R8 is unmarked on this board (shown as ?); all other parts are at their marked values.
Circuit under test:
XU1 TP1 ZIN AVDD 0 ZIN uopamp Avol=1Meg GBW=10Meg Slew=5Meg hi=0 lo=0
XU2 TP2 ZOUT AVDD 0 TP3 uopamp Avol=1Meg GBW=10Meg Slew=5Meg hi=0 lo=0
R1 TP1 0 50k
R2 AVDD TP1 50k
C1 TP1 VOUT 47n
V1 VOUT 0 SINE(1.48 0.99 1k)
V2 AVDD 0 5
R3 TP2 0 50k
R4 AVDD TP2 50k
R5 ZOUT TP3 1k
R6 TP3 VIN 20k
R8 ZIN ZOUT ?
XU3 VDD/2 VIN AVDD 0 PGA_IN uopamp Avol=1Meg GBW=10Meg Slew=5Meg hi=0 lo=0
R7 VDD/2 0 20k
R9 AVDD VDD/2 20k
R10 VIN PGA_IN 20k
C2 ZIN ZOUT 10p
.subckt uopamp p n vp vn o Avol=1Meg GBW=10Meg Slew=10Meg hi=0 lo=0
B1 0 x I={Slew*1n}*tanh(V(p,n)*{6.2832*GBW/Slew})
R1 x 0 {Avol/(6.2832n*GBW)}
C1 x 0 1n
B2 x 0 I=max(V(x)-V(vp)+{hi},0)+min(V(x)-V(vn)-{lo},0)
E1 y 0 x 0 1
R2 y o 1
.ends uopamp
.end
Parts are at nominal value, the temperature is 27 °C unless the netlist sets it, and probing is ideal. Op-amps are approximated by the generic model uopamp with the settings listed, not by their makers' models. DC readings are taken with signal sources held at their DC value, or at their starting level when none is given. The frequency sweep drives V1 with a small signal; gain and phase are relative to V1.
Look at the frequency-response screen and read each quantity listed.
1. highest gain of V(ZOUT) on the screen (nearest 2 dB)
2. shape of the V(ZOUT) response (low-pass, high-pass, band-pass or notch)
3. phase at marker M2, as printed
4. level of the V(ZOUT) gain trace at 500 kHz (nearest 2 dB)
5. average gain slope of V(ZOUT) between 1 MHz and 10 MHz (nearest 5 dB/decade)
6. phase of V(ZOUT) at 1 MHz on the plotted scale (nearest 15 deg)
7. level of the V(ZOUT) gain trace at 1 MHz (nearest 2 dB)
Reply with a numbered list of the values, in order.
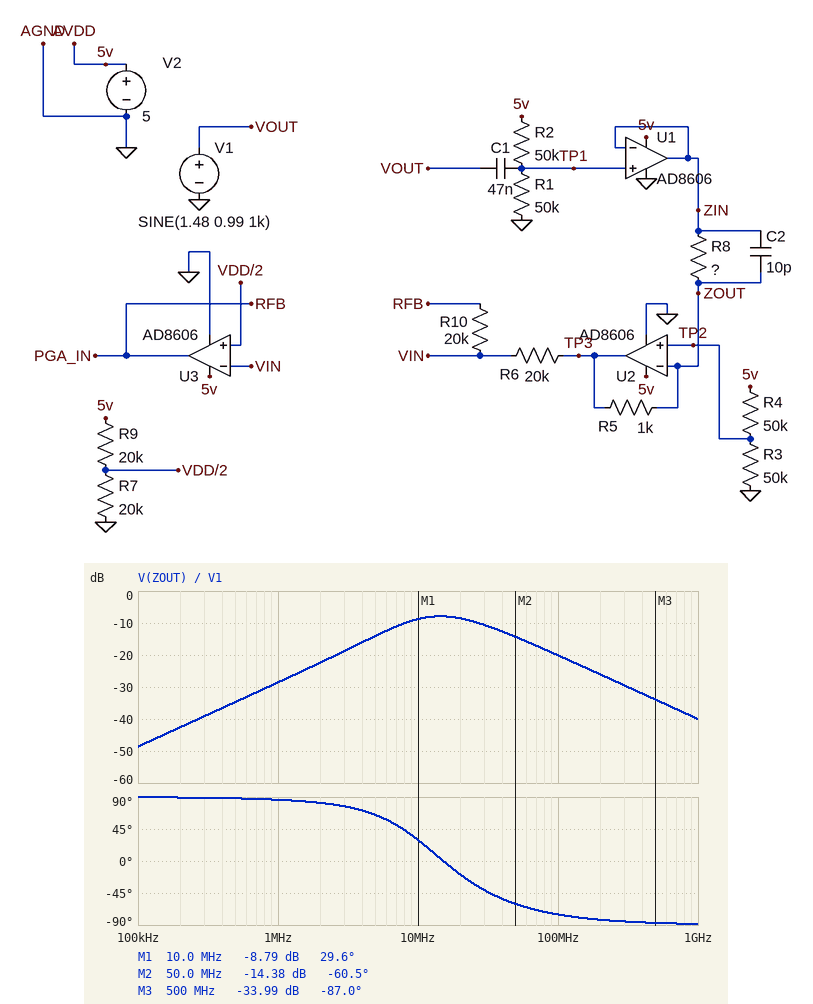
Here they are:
1. -8 dB
2. band-pass
3. -60.5 deg
4. -34 dB
5. 20 dB/decade
6. 90 deg
7. -28 dB
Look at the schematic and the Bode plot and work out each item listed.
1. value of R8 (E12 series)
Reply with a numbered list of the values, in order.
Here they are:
1. 2.7 kΩ
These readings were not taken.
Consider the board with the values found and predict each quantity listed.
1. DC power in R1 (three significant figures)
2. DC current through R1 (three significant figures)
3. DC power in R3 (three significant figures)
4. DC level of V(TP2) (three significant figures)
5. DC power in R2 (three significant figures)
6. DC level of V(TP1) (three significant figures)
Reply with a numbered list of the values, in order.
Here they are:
1. 125 µW
2. 50.0 µA
3. 125 µW
4. 2.50 V
5. 125 µW
6. 2.50 V
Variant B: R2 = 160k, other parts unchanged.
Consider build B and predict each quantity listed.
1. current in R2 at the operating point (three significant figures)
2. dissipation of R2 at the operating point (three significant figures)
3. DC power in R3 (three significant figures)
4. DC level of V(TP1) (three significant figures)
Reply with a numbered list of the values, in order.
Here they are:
1. 23.8 µA
2. 90.7 µW
3. 125 µW
4. 1.19 V
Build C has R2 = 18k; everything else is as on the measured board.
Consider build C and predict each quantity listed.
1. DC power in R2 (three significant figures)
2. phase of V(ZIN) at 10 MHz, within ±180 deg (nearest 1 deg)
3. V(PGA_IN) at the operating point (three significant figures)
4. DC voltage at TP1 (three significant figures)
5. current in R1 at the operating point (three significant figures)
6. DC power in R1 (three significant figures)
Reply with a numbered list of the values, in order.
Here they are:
1. 97.3 µW
2. -45 deg
3. 2.94 V
4. 3.68 V
5. 73.5 µA
6. 270 µW
